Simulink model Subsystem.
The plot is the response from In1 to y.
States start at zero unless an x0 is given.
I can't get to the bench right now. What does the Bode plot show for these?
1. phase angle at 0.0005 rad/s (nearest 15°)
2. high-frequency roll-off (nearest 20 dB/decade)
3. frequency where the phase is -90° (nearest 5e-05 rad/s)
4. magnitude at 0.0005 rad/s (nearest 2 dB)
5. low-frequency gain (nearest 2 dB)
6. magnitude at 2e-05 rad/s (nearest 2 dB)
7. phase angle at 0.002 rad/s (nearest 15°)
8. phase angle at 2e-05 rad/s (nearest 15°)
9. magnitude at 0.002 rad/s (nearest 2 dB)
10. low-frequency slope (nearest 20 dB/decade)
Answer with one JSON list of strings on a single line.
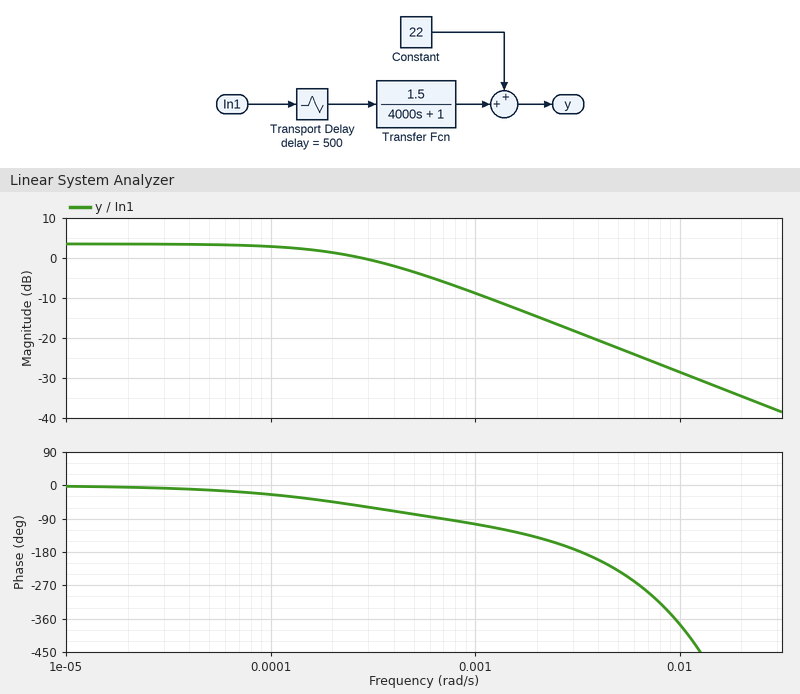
["-75°", "-20 dB/decade", "0.00070 rad/s", "-4 dB", "4 dB", "4 dB", "-135°", "0°", "-14 dB", "0 dB/decade"]
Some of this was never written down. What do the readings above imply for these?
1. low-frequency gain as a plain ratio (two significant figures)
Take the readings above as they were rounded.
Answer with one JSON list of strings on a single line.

["1.6"]
